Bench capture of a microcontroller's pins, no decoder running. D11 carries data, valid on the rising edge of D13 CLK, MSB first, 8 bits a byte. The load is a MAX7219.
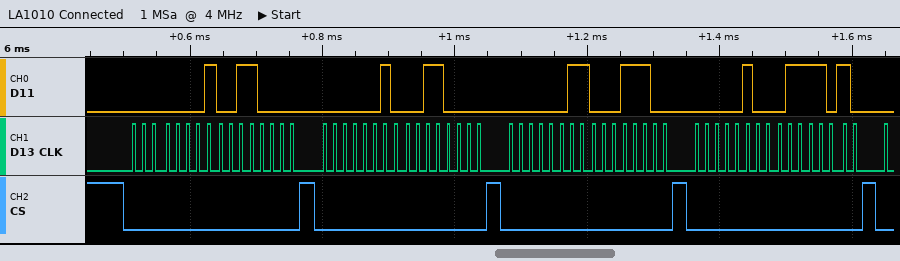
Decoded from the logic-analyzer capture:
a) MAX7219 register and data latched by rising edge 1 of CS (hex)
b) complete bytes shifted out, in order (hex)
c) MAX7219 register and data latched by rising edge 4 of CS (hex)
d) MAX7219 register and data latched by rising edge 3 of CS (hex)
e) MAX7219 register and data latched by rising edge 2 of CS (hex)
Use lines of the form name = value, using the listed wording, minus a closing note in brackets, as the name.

MAX7219 register and data latched by rising edge 1 of CS = register 0x1, data 0x30
complete bytes shifted out, in order = 01 30 02 30 03 1C 04 7A
MAX7219 register and data latched by rising edge 4 of CS = register 0x4, data 0x7A
MAX7219 register and data latched by rising edge 3 of CS = register 0x3, data 0x1C
MAX7219 register and data latched by rising edge 2 of CS = register 0x2, data 0x30
